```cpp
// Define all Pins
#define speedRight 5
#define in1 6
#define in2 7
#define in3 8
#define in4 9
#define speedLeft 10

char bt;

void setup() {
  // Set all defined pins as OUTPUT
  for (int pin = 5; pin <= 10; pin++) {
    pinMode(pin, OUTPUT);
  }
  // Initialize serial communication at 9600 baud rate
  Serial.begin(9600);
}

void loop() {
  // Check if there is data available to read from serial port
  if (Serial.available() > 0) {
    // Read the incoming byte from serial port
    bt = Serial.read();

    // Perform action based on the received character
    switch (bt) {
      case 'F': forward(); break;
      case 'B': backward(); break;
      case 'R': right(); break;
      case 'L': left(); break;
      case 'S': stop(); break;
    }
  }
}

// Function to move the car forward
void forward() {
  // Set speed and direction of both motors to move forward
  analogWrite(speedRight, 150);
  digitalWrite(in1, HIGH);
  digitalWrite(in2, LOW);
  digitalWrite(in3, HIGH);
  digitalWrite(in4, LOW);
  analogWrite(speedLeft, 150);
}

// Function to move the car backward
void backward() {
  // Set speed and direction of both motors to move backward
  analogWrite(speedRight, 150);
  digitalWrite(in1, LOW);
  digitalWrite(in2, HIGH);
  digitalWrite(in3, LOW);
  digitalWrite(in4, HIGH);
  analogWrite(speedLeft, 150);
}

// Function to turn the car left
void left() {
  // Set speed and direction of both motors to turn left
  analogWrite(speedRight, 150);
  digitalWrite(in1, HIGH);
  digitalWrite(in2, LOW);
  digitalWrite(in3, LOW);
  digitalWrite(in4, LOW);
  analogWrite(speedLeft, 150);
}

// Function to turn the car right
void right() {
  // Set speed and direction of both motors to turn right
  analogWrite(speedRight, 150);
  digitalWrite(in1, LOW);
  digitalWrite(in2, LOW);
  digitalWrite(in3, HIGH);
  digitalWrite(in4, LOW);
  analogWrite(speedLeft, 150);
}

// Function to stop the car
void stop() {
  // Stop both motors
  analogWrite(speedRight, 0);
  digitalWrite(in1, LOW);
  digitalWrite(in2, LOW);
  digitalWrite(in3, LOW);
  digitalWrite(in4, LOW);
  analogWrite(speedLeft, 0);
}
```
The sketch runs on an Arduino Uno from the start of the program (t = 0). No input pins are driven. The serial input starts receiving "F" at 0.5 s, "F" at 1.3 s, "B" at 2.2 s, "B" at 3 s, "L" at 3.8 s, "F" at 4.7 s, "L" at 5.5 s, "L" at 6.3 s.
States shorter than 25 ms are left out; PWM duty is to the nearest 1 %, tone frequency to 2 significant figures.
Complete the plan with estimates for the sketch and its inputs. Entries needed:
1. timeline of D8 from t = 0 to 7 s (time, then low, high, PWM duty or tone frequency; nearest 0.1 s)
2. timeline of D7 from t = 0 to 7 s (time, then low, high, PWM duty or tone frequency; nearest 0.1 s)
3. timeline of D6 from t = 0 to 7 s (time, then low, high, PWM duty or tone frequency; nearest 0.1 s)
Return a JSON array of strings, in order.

["0 s low; 0.5 s high; 2.2 s low; 4.7 s high; 5.5 s low", "0 s low; 2.2 s high; 3.8 s low", "0 s low; 0.5 s high; 2.2 s low; 3.8 s high"]
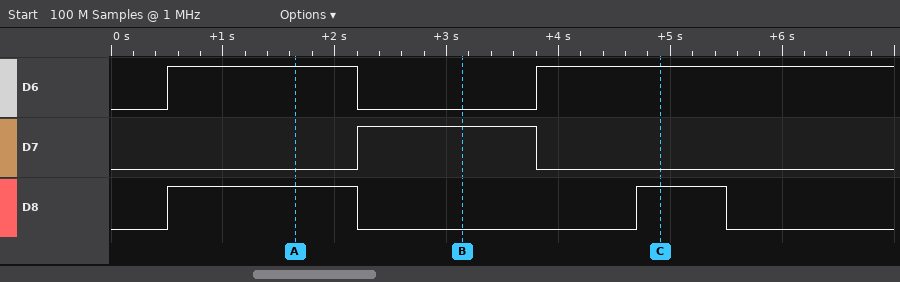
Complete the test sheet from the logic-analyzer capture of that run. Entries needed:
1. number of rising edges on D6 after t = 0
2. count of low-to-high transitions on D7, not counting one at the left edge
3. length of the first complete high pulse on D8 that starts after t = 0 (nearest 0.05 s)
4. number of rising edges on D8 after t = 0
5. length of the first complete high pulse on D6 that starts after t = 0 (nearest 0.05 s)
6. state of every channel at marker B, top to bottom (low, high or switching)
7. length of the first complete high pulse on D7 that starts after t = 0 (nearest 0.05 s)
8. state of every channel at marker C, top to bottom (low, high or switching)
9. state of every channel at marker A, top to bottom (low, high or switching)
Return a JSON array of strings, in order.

["2", "1", "1.70 s", "2", "1.70 s", "D6 low, D7 high, D8 low", "1.60 s", "D6 high, D7 low, D8 high", "D6 high, D7 low, D8 high"]
